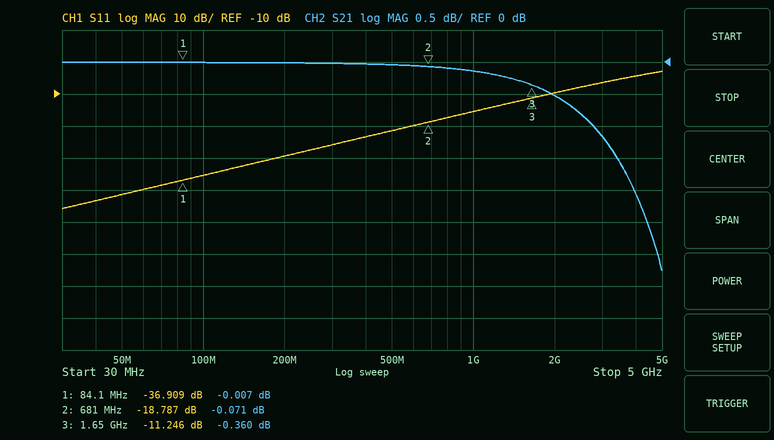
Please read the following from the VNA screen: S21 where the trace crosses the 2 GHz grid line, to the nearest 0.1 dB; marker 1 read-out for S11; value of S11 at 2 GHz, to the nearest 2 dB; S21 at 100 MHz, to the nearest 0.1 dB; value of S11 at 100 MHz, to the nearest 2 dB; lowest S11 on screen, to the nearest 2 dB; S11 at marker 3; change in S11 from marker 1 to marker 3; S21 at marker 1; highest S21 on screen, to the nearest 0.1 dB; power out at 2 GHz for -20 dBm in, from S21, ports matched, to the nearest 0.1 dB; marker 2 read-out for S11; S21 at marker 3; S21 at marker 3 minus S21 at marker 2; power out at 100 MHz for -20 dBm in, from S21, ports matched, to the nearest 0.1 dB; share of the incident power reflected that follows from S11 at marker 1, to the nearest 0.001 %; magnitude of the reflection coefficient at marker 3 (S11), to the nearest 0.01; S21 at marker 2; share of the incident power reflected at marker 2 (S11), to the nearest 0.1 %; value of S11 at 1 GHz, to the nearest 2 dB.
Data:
-0.5 dB
-36.909 dB
-10 dB
0.0 dB
-36 dB
-46 dB
-11.246 dB
25.663 dB
-0.007 dB
0.0 dB
-20.5 dBm
-18.787 dB
-0.360 dB
-0.289 dB
-20.0 dBm
0.020 %
0.27
-0.071 dB
1.3 %
-16 dB
